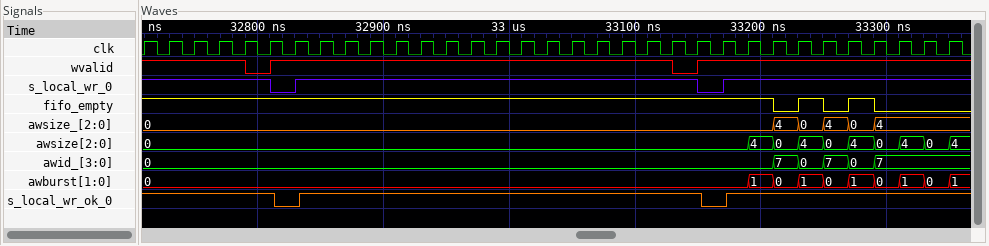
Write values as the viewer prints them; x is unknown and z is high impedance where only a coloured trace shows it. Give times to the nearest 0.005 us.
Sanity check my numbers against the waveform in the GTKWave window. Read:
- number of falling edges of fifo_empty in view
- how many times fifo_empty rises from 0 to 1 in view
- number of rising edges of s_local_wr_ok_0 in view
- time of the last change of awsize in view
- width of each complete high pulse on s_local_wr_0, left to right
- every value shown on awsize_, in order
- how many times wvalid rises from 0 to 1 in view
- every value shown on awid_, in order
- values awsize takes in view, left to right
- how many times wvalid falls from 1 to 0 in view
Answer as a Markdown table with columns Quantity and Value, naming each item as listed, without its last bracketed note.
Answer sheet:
| Quantity | Value |
|---|---|
| number of falling edges of fifo_empty in view | 3 |
| how many times fifo_empty rises from 0 to 1 in view | 2 |
| number of rising edges of s_local_wr_ok_0 in view | 2 |
| time of the last change of awsize in view | 33.35 us |
| width of each complete high pulse on s_local_wr_0, left to right | 0.32 us |
| every value shown on awsize_, in order | 0, 4, 0, 4, 0, 4 |
| how many times wvalid rises from 0 to 1 in view | 2 |
| every value shown on awid_, in order | 0, 7, 0, 7, 0, 7 |
| values awsize takes in view, left to right | 0, 4, 0, 4, 0, 4, 0, 4, 0, 4 |
| how many times wvalid falls from 1 to 0 in view | 2 |
